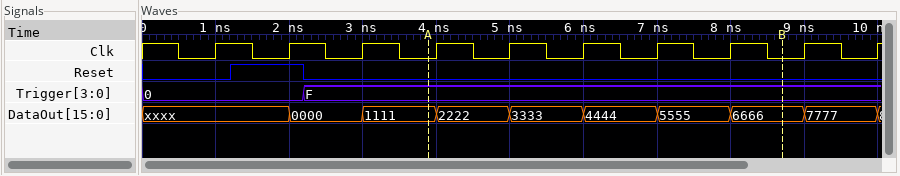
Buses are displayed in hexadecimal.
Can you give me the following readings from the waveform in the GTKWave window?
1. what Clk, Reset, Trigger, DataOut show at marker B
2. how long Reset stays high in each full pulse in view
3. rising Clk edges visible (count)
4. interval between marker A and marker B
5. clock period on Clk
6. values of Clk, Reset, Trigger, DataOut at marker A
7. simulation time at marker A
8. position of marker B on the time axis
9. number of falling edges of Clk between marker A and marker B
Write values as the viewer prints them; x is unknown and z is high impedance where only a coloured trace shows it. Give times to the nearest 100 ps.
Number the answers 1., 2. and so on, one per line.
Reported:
1. Clk=0, Reset=0, Trigger=F, DataOut=6666
2. 1000 ps
3. 10
4. 4800 ps
5. 1000 ps
6. Clk=0, Reset=0, Trigger=F, DataOut=1111
7. 3900 ps
8. 8700 ps
9. 5
